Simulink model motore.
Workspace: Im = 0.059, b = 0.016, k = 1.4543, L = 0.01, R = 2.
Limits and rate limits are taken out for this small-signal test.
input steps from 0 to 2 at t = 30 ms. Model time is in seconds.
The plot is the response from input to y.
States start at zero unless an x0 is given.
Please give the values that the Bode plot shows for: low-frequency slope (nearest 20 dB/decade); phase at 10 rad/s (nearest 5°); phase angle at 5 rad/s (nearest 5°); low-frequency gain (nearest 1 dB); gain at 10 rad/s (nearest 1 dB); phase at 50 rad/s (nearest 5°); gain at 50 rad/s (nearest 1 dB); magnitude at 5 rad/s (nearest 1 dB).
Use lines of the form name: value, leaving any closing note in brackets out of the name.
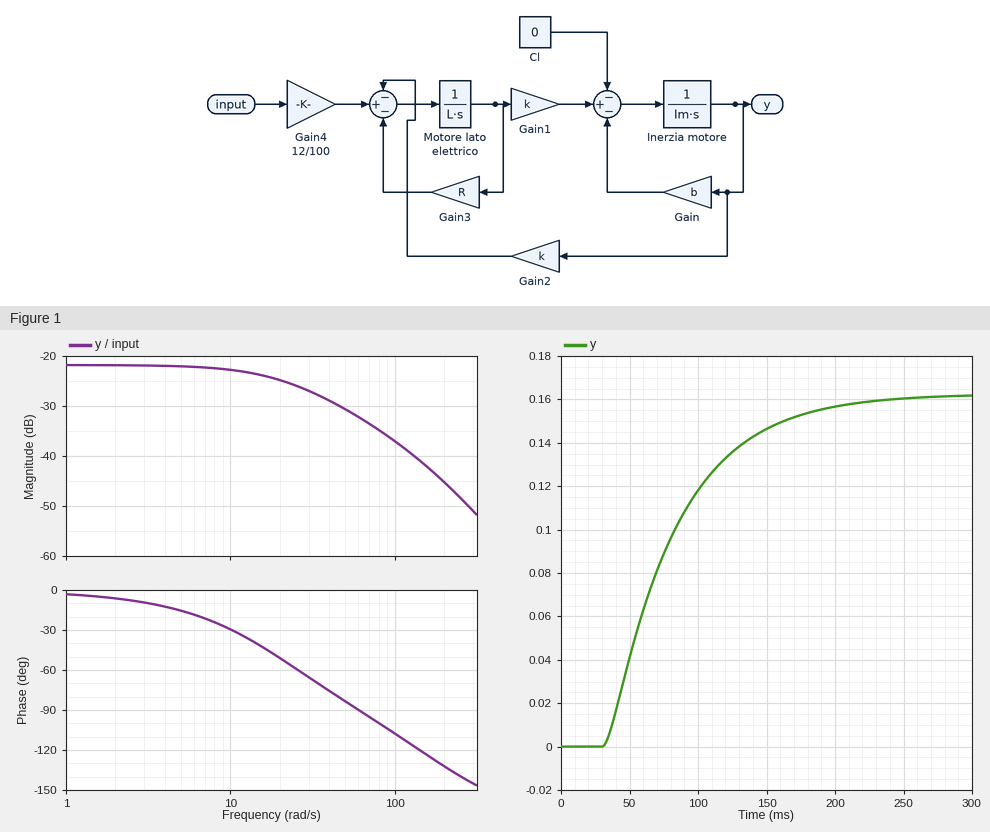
low-frequency slope: 0 dB/decade
phase at 10 rad/s: -30°
phase angle at 5 rad/s: -15°
low-frequency gain: -22 dB
gain at 10 rad/s: -23 dB
phase at 50 rad/s: -85°
gain at 50 rad/s: -31 dB
magnitude at 5 rad/s: -22 dB
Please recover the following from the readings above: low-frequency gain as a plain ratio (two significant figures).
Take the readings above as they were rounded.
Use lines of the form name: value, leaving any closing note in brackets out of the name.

low-frequency gain as a plain ratio: 0.079
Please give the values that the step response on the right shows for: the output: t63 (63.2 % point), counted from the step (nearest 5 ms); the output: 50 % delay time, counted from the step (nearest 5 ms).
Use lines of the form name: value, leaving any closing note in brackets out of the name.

the output: t63 (63.2 % point), counted from the step: 55 ms
the output: 50 % delay time, counted from the step: 40 ms
